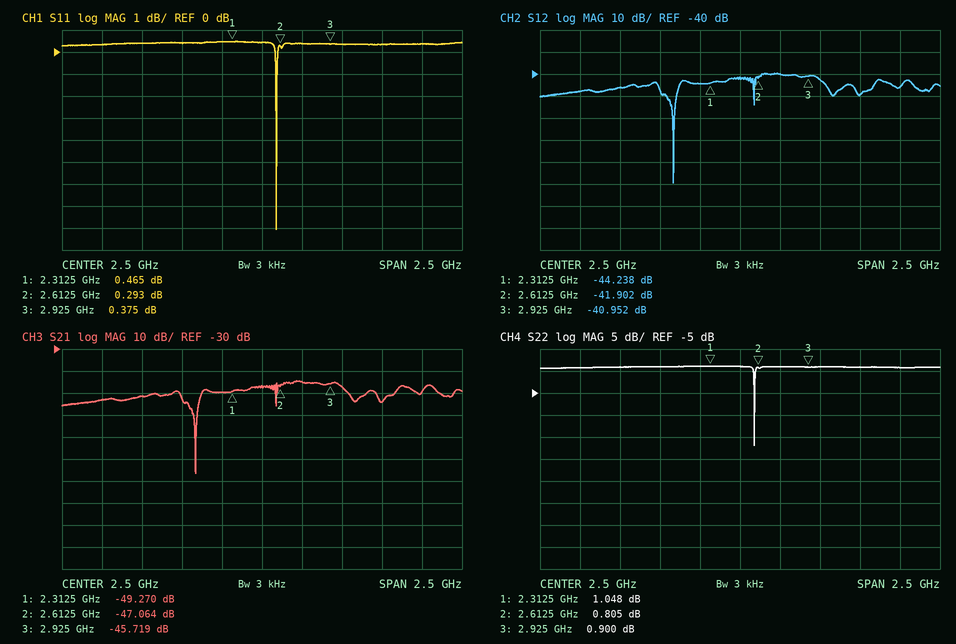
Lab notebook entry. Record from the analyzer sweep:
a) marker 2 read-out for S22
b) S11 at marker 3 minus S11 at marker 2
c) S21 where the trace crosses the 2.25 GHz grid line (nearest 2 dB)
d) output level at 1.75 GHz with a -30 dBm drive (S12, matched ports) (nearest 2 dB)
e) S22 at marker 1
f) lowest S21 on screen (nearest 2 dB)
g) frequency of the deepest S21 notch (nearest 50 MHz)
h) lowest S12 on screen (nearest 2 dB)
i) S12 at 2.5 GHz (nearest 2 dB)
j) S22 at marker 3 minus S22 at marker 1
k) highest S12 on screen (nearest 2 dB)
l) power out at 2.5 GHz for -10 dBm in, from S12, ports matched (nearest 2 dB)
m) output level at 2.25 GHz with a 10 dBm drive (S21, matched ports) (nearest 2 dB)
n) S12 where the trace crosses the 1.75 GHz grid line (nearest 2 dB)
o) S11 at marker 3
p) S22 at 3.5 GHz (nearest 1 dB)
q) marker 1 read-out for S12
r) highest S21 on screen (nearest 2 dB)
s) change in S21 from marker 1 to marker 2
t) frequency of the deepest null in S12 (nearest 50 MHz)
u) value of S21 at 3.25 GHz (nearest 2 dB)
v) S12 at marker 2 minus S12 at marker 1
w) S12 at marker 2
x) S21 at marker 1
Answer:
0.805 dB
0.082 dB
-50 dB
-76 dBm
1.048 dB
-86 dB
2.10 GHz
-90 dB
-42 dB
-0.148 dB
-40 dB
-52 dBm
-40 dBm
-46 dB
0.375 dB
1 dB
-44.238 dB
-44 dB
2.206 dB
2.10 GHz
-54 dB
2.336 dB
-41.902 dB
-49.270 dB
